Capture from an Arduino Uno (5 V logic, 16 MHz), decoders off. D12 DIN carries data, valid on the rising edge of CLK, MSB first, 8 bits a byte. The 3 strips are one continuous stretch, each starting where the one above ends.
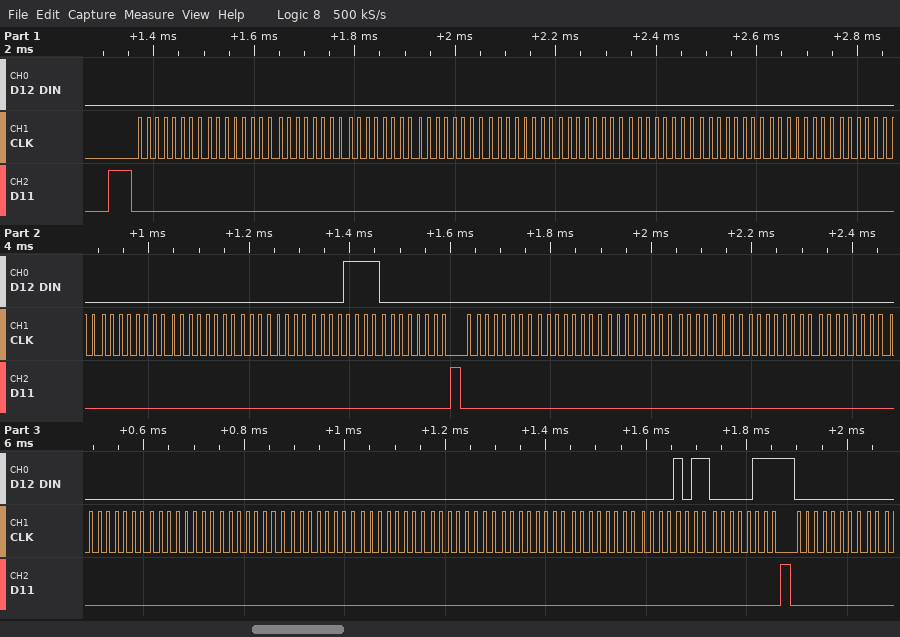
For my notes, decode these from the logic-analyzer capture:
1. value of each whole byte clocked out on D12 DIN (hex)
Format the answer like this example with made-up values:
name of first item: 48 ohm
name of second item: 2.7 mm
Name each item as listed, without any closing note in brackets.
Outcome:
value of each whole byte clocked out on D12 DIN: 0x00 0x00 0x00 0x00 0x00 0x00 0x00 0x00 0x00 0x00 0x00 0x00 0x00 0x00 0x0F 0x00 0x00 0x00 0x00 0x00 0x00 0x00 0x00 0x00 0x00 0x00 0x00 0x00 0x00 0x00 0x0B 0x07 0x00
